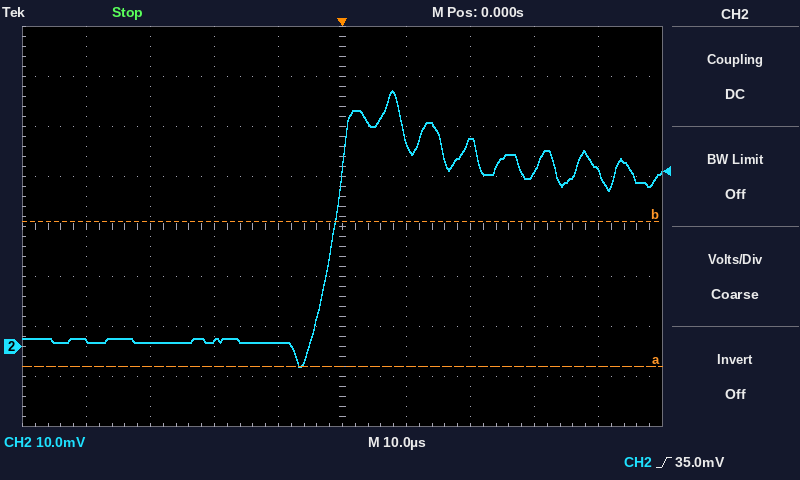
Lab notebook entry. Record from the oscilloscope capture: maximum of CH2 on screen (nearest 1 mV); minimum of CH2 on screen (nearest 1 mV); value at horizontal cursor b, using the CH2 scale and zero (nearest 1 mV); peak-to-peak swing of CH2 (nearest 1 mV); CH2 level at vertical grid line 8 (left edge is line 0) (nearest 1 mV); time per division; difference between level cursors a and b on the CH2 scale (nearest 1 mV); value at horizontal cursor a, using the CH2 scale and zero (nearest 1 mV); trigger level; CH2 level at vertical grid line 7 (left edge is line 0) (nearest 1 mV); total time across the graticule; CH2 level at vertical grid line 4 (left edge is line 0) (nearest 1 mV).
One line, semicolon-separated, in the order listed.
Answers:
51 mV; -4 mV; 25 mV; 55 mV; 35 mV; 10 µs; 29 mV; -4 mV; 35.0 mV; 41 mV; 100 µs; 1 mV
